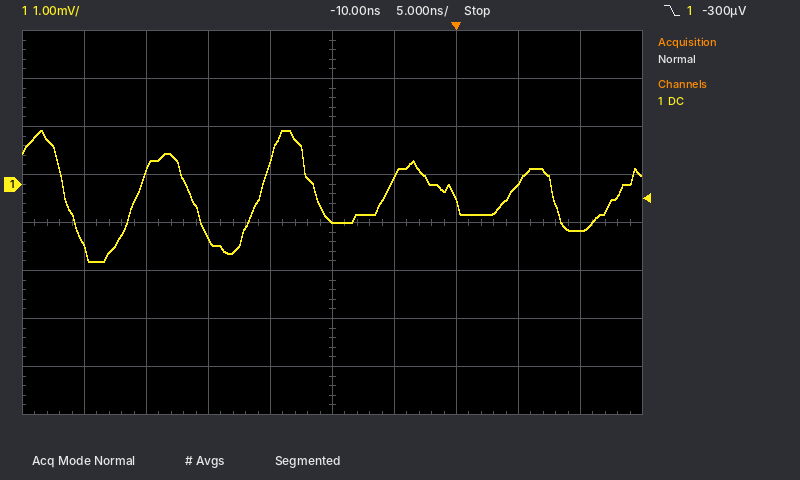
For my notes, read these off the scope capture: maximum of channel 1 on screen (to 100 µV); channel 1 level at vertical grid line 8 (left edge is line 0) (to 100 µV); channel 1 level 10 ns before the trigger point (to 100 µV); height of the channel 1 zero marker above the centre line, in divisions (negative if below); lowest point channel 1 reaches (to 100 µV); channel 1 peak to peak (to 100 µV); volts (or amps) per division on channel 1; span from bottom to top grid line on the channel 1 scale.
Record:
1.1 mV
0.0 mV
-800 µV
+0.8 div
-1.6 mV
2.7 mV
1 mV
8 mV
